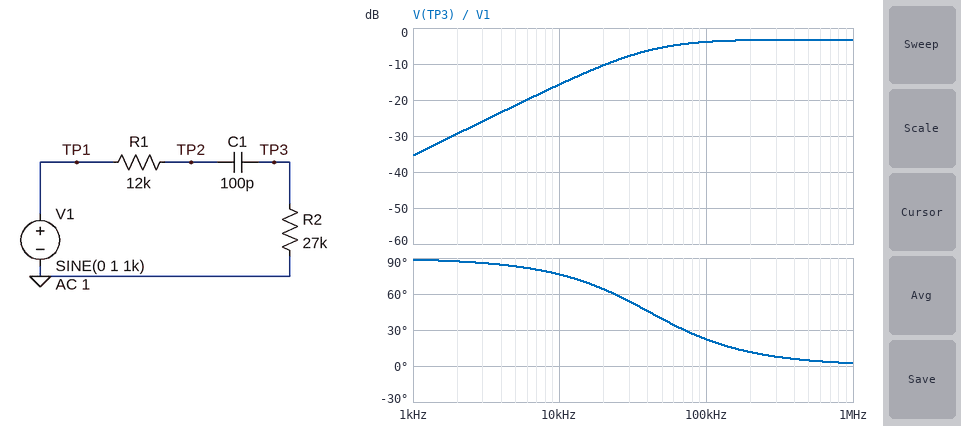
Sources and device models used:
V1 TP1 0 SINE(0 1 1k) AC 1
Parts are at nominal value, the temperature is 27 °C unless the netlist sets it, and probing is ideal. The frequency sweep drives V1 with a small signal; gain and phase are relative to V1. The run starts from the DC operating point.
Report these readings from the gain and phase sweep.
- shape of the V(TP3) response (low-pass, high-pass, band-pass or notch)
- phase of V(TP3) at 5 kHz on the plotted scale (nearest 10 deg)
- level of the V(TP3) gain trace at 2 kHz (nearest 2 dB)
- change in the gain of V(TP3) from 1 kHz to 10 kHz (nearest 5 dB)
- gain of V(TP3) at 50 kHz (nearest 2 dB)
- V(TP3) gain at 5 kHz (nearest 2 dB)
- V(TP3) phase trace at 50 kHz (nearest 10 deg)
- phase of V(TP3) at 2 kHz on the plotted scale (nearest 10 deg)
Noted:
high-pass
80 deg
-30 dB
20 dB
-6 dB
-22 dB
40 deg
90 deg
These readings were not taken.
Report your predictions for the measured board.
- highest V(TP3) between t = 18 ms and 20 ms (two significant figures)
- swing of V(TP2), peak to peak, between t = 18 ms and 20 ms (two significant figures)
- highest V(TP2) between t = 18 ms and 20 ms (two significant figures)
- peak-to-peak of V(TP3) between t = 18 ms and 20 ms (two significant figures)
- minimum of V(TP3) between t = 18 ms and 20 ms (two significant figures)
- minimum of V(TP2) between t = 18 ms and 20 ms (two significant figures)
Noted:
17 mV
2.0 V
1.0 V
34 mV
-17 mV
-1.0 V
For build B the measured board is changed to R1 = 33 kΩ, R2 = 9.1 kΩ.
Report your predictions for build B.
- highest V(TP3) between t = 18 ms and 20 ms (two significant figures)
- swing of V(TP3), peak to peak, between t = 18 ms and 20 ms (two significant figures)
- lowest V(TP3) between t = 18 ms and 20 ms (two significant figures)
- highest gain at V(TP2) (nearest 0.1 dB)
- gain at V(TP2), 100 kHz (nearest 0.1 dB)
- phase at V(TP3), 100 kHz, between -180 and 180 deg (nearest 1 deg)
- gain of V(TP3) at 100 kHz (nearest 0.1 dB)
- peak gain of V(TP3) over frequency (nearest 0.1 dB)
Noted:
5.7 mV
11 mV
-5.7 mV
0 dB
-7.8 dB
21 deg
-13.9 dB
-13.3 dB
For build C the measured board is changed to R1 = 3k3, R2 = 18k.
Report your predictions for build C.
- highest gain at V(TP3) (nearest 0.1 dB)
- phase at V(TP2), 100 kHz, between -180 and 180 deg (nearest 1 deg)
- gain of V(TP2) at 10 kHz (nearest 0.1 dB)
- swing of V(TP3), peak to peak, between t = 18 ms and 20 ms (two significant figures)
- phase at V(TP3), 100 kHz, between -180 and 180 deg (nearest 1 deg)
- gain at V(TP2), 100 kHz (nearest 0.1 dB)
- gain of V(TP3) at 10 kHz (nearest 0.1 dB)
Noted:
-1.5 dB
-5 deg
0 dB
23 mV
37 deg
-0.9 dB
-19.0 dB
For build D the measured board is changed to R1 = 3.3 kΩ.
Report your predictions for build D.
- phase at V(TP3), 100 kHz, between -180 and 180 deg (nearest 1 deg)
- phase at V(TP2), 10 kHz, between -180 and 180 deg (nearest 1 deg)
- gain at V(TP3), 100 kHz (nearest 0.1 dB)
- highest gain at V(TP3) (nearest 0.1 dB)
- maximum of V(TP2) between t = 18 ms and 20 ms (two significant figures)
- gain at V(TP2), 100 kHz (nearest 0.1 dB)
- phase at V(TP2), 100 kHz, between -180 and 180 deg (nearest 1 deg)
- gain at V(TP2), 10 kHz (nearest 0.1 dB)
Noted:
28 deg
-1 deg
-2.1 dB
-1.0 dB
1.0 V
-0.8 dB
-3 deg
0 dB
